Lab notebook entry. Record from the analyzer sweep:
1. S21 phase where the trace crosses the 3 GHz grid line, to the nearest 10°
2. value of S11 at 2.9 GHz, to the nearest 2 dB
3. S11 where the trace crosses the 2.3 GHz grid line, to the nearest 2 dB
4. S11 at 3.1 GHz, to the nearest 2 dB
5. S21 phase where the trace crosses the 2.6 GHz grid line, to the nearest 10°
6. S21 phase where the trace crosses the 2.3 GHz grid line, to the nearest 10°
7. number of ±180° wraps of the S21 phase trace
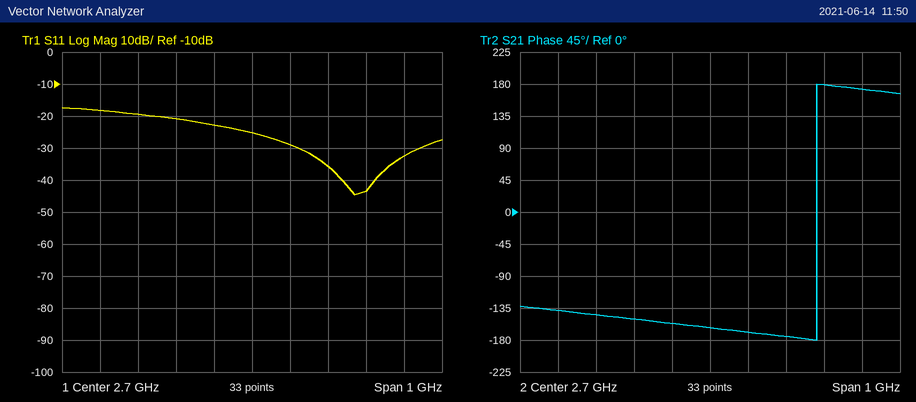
180°
-36 dB
-18 dB
-32 dB
-160°
-140°
1
